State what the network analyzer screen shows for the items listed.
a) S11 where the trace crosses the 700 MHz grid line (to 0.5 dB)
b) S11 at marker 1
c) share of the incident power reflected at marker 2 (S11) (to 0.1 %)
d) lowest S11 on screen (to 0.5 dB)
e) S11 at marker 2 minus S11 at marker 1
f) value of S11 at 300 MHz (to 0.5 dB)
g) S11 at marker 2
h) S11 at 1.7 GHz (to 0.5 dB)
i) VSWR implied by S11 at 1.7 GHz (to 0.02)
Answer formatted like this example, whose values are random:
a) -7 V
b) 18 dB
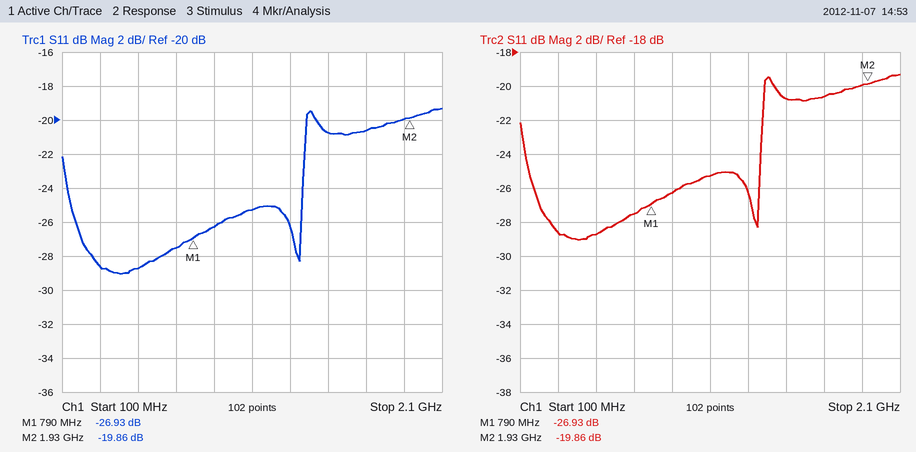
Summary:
a) -27.5 dB
b) -26.93 dB
c) 1.0 %
d) -29.0 dB
e) 7.07 dB
f) -28.5 dB
g) -19.86 dB
h) -20.5 dB
i) 1.20
